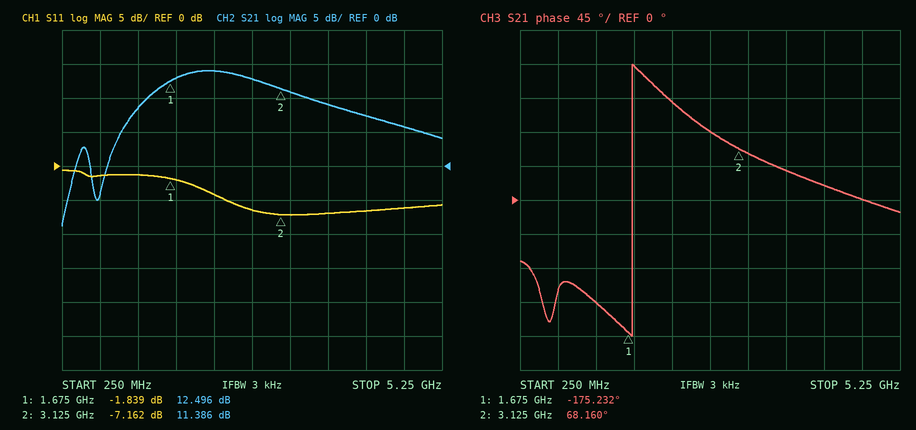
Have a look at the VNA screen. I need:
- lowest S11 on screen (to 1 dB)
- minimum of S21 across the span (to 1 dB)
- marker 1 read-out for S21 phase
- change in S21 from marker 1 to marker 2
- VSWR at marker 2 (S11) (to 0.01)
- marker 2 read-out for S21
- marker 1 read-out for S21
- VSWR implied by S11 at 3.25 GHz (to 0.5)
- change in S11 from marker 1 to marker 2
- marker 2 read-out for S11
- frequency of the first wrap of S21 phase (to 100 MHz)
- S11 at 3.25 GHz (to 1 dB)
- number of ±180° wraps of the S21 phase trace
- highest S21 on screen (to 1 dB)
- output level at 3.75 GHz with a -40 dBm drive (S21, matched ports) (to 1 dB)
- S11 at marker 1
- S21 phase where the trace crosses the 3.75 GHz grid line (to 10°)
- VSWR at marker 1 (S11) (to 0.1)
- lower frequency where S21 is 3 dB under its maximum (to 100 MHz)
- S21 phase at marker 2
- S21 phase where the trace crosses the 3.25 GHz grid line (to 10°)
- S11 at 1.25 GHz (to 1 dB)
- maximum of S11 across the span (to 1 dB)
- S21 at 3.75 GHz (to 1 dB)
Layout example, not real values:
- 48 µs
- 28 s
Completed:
- -7 dB
- -9 dB
- -175.232°
- -1.110 dB
- 2.56
- 11.386 dB
- 12.496 dB
- 2.5
- -5.323 dB
- -7.162 dB
- 1.7 GHz
- -7 dB
- 1
- 14 dB
- -31 dBm
- -1.839 dB
- 40°
- 9.5
- 1.5 GHz
- 68.160°
- 60°
- -1 dB
- -1 dB
- 9 dB
